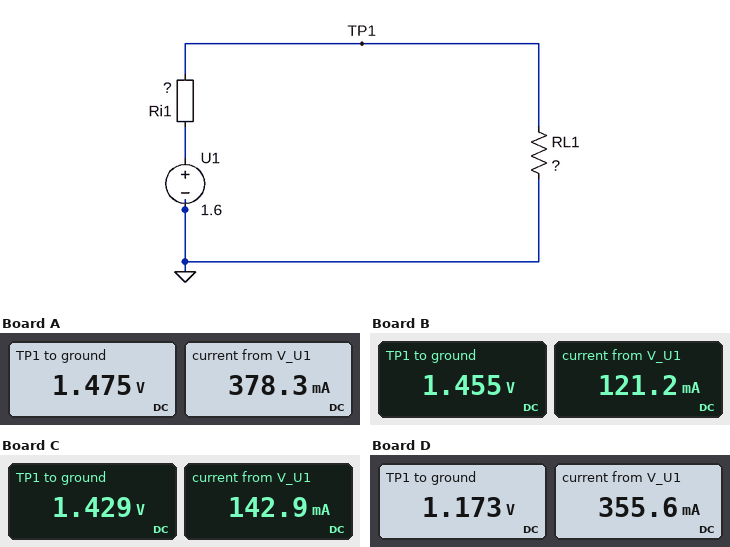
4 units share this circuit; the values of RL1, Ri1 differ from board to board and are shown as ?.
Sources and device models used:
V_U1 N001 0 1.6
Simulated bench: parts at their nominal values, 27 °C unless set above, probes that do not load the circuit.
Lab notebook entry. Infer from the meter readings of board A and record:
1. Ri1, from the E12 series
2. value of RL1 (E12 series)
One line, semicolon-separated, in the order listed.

0.33 Ω; 3.9 Ω
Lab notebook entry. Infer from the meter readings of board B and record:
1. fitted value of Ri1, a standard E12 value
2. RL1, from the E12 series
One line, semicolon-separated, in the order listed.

1.2 Ω; 12 Ω
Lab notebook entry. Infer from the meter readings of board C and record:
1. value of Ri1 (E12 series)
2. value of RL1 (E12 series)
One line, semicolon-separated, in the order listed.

1.2 Ω; 10 Ω
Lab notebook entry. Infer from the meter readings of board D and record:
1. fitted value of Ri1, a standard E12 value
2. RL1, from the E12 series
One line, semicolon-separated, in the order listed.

1.2 Ω; 3.3 Ω
